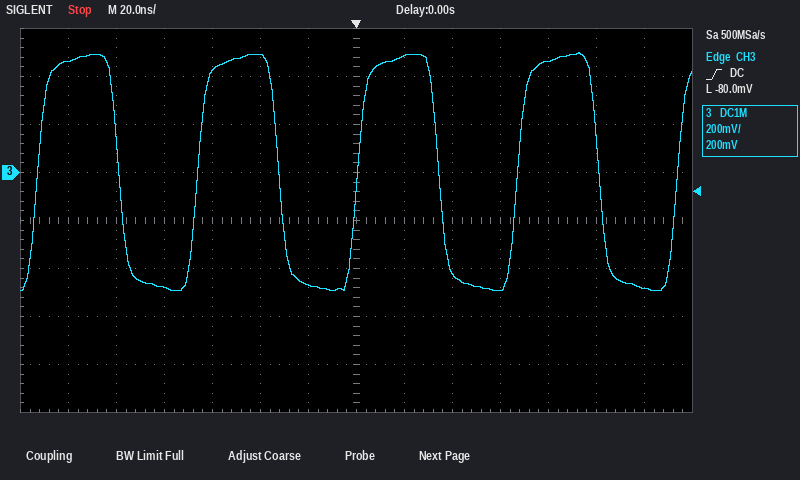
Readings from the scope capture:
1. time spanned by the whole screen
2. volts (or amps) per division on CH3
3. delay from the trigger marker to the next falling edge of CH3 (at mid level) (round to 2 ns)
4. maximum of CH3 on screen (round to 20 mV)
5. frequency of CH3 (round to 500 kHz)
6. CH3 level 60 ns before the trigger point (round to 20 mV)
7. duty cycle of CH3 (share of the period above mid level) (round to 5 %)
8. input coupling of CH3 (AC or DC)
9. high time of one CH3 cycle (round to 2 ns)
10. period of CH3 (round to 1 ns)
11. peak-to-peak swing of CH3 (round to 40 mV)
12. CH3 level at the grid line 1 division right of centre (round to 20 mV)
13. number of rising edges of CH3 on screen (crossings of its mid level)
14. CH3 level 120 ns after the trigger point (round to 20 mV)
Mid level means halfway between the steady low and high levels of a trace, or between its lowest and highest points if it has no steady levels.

280 ns
200 mV
34 ns
500 mV
15.0 MHz
420 mV
50 %
DC
34 ns
67 ns
1.00 V
480 mV
5
-480 mV
